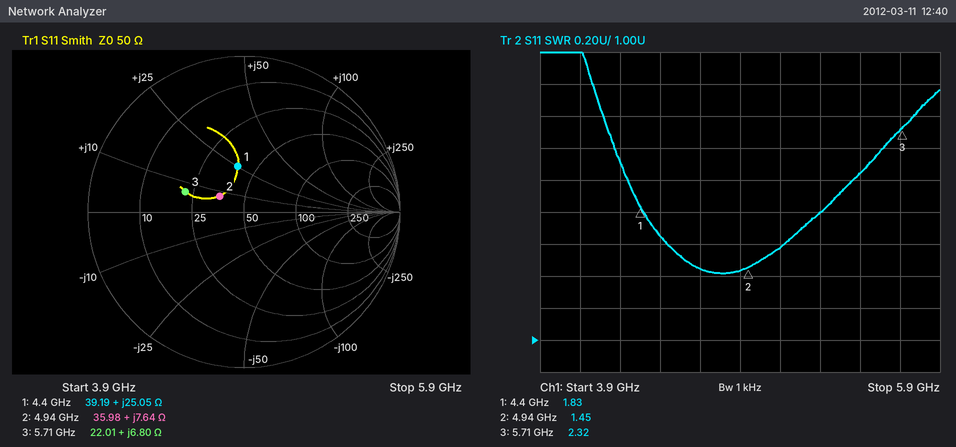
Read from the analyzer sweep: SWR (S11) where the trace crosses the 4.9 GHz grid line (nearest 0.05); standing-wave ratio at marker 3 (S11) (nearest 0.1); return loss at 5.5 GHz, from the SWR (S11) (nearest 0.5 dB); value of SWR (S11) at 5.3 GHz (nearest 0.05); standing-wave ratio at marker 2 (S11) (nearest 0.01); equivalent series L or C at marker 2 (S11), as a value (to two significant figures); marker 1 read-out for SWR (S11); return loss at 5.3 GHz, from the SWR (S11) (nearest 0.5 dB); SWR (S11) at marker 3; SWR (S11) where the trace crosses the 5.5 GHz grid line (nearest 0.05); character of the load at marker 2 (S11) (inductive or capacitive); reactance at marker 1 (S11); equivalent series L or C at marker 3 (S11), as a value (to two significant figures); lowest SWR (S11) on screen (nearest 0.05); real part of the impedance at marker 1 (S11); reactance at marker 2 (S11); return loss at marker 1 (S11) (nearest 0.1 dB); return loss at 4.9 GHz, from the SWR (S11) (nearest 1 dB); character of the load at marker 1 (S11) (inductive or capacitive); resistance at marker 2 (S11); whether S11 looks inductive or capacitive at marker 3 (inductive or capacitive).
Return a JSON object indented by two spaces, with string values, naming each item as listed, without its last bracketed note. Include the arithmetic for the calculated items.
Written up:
{
  "SWR (S11) where the trace crosses the 4.9 GHz grid line": "1.45",
  "standing-wave ratio at marker 3 (S11)": "2.3",
  "return loss at 5.5 GHz, from the SWR (S11)": "−20 log10((2.05 − 1)/(2.05 + 1)) ≈ 9.26 dB, so 9.5 dB to the nearest 0.5 dB",
  "value of SWR (S11) at 5.3 GHz": "1.80",
  "standing-wave ratio at marker 2 (S11)": "1.45",
  "equivalent series L or C at marker 2 (S11), as a value": "L = 7.64 Ω/(2π × 4.94 GHz) ≈ 246 pH, so 250 pH to two significant figures",
  "marker 1 read-out for SWR": "1.83",
  "return loss at 5.3 GHz, from the SWR (S11)": "−20 log10((1.8 − 1)/(1.8 + 1)) ≈ 10.9 dB, so 11.0 dB to the nearest 0.5 dB",
  "SWR (S11) at marker 3": "2.32",
  "SWR (S11) where the trace crosses the 5.5 GHz grid line": "2.05",
  "character of the load at marker 2 (S11)": "inductive",
  "reactance at marker 1": "+25.05 Ω",
  "equivalent series L or C at marker 3 (S11), as a value": "L = 6.8 Ω/(2π × 5.71 GHz) ≈ 190 pH",
  "lowest SWR (S11) on screen": "1.40",
  "real part of the impedance at marker 1": "39.19 Ω",
  "reactance at marker 2": "+7.64 Ω",
  "return loss at marker 1 (S11)": "10.6 dB",
  "return loss at 4.9 GHz, from the SWR (S11)": "−20 log10((1.45 − 1)/(1.45 + 1)) ≈ 15 dB",
  "character of the load at marker 1 (S11)": "inductive",
  "resistance at marker 2": "35.98 Ω",
  "whether S11 looks inductive or capacitive at marker 3": "inductive"
}
